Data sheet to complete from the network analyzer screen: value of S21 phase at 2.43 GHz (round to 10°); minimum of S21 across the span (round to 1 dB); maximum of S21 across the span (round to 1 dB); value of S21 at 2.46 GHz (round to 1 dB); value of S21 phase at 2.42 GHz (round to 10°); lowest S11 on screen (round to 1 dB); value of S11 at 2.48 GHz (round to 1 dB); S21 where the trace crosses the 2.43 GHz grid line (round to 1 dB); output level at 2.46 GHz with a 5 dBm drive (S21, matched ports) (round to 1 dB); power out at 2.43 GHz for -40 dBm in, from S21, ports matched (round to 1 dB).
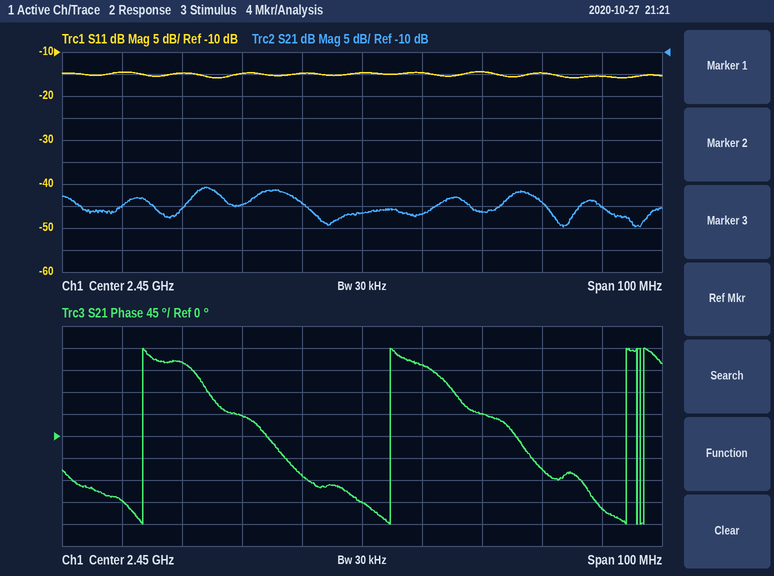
40°
-50 dB
-41 dB
-47 dB
150°
-16 dB
-15 dB
-45 dB
-42 dBm
-85 dBm
